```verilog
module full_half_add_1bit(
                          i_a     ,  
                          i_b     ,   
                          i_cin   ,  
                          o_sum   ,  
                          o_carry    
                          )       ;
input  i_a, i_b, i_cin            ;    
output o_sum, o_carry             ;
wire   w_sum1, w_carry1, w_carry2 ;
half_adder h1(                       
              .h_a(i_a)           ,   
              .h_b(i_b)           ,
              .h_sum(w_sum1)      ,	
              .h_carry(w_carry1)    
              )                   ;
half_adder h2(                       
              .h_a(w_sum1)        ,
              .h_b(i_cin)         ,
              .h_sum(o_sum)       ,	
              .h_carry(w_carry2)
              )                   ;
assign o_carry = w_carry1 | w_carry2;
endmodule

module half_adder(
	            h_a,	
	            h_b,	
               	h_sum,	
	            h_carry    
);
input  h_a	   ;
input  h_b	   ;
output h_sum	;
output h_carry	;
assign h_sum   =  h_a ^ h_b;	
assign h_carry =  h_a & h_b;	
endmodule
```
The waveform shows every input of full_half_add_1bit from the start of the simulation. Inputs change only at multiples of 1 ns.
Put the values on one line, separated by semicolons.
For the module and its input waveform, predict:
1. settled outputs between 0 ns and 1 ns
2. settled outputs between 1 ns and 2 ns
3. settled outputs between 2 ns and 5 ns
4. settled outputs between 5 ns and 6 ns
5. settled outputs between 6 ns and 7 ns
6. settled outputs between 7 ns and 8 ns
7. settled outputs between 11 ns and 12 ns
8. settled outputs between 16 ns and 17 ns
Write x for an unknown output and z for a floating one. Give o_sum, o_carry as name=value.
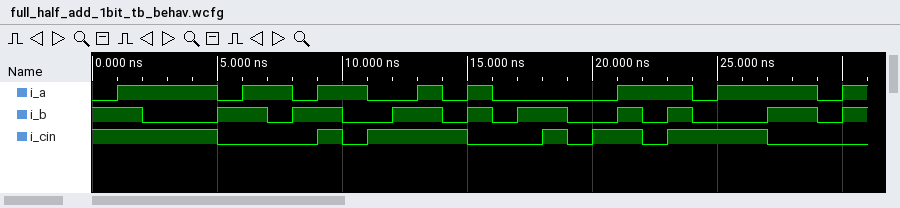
o_sum=0, o_carry=1; o_sum=1, o_carry=1; o_sum=0, o_carry=1; o_sum=1, o_carry=0; o_sum=0, o_carry=1; o_sum=1, o_carry=0; o_sum=1, o_carry=0; o_sum=0, o_carry=0
